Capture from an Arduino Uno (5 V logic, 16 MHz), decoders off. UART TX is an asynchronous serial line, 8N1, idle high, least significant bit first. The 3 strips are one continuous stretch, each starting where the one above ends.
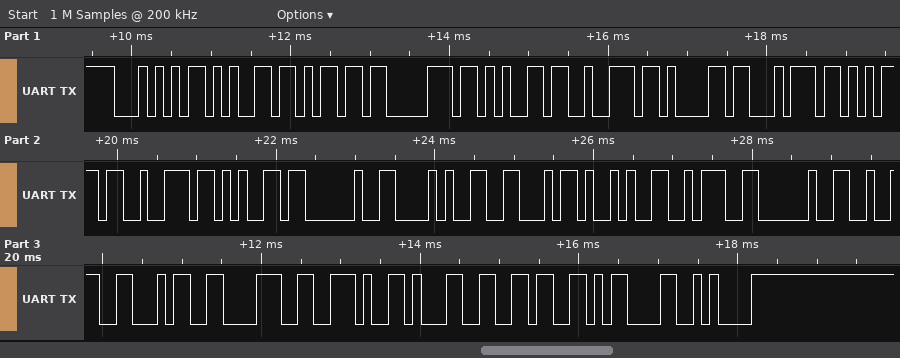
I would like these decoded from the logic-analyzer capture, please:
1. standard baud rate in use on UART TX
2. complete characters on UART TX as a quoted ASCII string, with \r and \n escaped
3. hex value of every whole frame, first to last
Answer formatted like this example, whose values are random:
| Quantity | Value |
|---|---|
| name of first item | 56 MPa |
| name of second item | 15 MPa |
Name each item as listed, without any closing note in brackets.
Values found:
| Quantity | Value |
|---|---|
| standard baud rate in use on UART TX | 9600 baud |
| complete characters on UART TX as a quoted ASCII string, with \r and \n escaped | "Temperature (F): 248.16\r\n" |
| hex value of every whole frame, first to last | 54 65 6D 70 65 72 61 74 75 72 65 20 28 46 29 3A 20 32 34 38 2E 31 36 0D 0A |
